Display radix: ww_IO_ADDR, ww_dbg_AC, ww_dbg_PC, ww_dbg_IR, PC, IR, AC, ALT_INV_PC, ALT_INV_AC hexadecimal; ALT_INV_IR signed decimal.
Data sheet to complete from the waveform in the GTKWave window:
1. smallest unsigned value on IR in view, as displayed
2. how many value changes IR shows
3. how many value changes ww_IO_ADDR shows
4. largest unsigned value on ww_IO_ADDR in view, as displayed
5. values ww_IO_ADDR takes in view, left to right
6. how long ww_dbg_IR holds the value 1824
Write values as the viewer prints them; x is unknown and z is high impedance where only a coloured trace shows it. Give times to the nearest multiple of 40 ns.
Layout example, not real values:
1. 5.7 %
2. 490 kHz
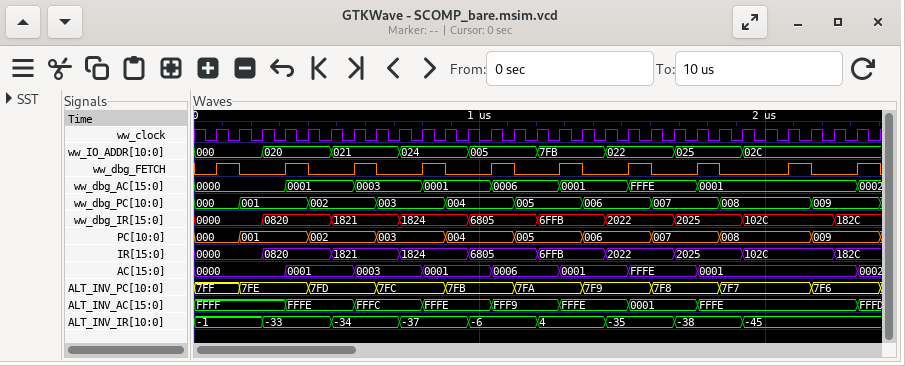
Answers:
1. 0000
2. 9
3. 8
4. 7FB
5. 000, 020, 021, 024, 005, 7FB, 022, 025, 02C
6. 240 ns
